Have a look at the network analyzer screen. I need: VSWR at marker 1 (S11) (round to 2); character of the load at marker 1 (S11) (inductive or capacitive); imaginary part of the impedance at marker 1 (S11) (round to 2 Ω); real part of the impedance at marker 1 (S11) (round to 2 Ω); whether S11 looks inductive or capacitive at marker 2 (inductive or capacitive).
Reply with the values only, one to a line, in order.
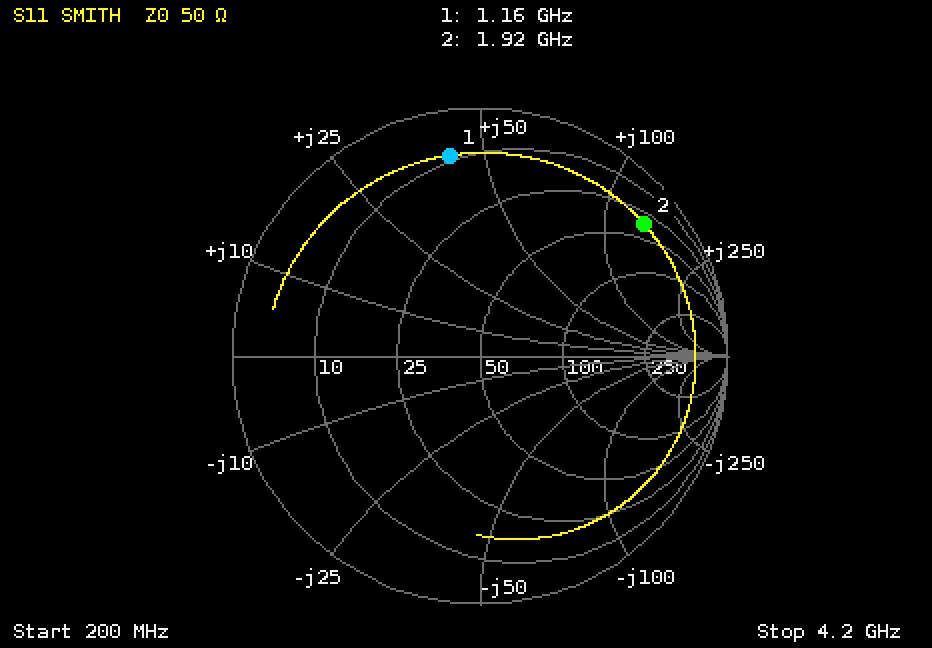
10
inductive
+42 Ω
8 Ω
inductive
